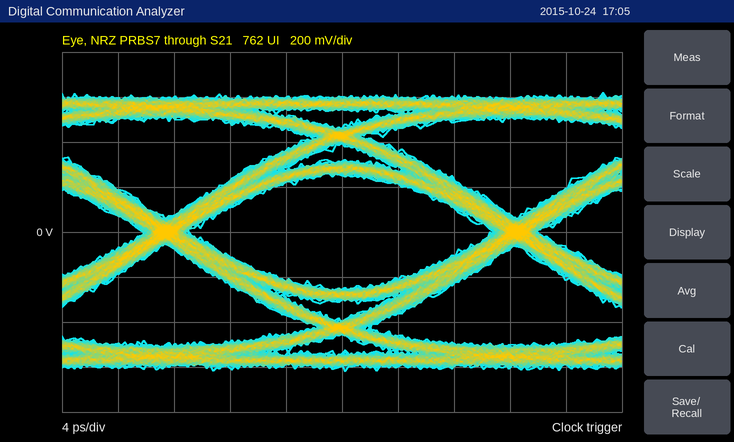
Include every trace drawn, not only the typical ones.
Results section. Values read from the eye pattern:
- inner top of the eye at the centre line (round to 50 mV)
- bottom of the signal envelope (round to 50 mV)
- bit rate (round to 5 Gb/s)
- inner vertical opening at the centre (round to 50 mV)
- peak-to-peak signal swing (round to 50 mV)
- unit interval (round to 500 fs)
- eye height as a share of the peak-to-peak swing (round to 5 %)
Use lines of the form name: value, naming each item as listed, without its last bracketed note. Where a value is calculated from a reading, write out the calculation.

inner top of the eye at the centre line: 250 mV
bottom of the signal envelope: -600 mV
bit rate: 40 Gb/s
inner vertical opening at the centre: 500 mV
peak-to-peak signal swing: 1.25 V
unit interval: 25.0 ps
eye height as a share of the peak-to-peak swing: 500 mV / 1.25 V ≈ 40 %
